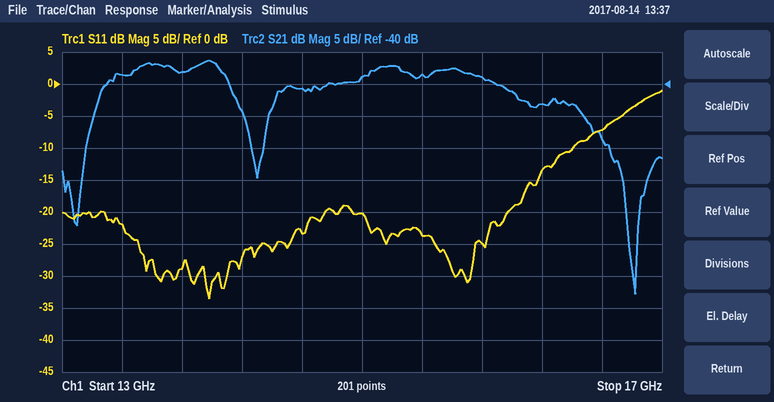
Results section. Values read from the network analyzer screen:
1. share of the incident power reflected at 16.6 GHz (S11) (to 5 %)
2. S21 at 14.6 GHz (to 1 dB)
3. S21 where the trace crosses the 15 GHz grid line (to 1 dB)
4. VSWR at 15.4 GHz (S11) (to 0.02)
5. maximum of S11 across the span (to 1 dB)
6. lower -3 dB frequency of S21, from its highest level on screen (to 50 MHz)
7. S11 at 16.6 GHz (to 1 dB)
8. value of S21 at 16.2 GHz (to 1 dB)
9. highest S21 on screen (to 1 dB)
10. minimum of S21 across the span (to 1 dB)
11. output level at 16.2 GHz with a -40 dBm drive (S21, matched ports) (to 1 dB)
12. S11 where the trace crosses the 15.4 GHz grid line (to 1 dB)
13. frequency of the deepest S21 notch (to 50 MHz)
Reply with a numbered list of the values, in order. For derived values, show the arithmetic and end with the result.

1. 10^(-7/10) ≈ 20 %
2. -41 dB
3. -39 dB
4. |Γ| = 10^(-24/20) = 0.0631; VSWR = (1 + 0.0631)/(1 − 0.0631) ≈ 1.13, so 1.14 to the nearest 0.02
5. -1 dB
6. 13.35 GHz
7. -7 dB
8. -43 dB
9. -36 dB
10. -73 dB
11. -40 dBm + (-43 dB) = -83 dBm
12. -24 dB
13. 16.80 GHz
